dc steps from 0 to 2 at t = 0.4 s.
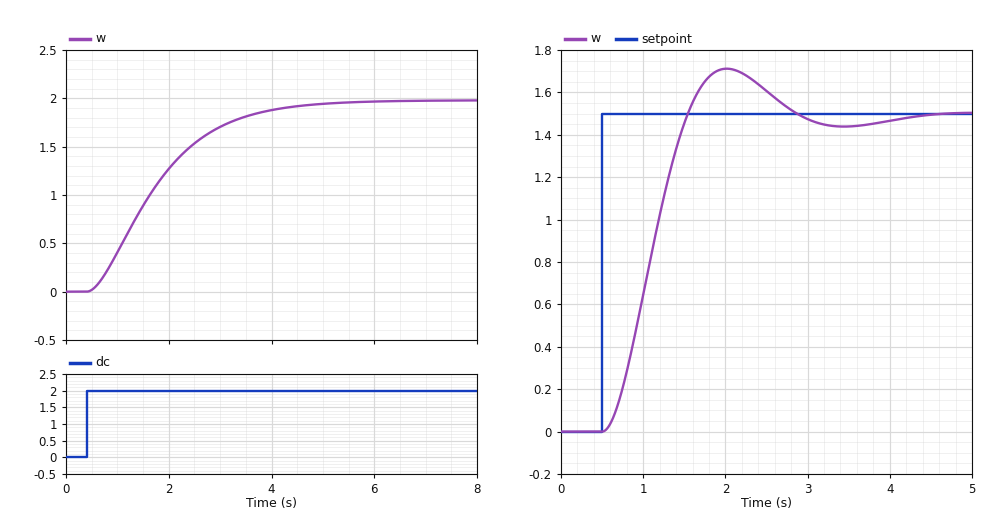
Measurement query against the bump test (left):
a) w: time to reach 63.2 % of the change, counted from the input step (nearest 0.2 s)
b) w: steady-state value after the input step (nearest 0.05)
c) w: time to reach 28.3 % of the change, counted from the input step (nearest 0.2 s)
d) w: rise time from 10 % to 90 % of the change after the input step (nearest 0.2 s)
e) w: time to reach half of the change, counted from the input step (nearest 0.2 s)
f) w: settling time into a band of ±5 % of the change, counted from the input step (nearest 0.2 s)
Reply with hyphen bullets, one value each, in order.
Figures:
- 1.6 s
- 2.00
- 0.8 s
- 2.6 s
- 1.2 s
- 3.6 s
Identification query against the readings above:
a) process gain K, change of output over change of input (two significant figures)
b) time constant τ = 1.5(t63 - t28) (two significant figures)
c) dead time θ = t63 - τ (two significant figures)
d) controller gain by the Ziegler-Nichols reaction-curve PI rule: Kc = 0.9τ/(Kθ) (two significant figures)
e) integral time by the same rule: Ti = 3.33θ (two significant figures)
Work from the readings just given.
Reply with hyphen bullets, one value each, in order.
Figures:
- 1.0
- 1.2 s
- 0.40 s
- 2.7
- 1.3 s
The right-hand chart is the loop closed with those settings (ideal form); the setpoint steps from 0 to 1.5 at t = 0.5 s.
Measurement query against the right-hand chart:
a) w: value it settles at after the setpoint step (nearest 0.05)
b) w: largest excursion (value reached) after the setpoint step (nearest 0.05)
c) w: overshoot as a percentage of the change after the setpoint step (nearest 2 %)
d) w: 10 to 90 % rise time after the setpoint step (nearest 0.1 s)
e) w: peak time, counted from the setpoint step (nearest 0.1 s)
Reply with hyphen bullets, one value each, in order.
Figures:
- 1.50
- 1.70
- 14 %
- 0.7 s
- 1.5 s
